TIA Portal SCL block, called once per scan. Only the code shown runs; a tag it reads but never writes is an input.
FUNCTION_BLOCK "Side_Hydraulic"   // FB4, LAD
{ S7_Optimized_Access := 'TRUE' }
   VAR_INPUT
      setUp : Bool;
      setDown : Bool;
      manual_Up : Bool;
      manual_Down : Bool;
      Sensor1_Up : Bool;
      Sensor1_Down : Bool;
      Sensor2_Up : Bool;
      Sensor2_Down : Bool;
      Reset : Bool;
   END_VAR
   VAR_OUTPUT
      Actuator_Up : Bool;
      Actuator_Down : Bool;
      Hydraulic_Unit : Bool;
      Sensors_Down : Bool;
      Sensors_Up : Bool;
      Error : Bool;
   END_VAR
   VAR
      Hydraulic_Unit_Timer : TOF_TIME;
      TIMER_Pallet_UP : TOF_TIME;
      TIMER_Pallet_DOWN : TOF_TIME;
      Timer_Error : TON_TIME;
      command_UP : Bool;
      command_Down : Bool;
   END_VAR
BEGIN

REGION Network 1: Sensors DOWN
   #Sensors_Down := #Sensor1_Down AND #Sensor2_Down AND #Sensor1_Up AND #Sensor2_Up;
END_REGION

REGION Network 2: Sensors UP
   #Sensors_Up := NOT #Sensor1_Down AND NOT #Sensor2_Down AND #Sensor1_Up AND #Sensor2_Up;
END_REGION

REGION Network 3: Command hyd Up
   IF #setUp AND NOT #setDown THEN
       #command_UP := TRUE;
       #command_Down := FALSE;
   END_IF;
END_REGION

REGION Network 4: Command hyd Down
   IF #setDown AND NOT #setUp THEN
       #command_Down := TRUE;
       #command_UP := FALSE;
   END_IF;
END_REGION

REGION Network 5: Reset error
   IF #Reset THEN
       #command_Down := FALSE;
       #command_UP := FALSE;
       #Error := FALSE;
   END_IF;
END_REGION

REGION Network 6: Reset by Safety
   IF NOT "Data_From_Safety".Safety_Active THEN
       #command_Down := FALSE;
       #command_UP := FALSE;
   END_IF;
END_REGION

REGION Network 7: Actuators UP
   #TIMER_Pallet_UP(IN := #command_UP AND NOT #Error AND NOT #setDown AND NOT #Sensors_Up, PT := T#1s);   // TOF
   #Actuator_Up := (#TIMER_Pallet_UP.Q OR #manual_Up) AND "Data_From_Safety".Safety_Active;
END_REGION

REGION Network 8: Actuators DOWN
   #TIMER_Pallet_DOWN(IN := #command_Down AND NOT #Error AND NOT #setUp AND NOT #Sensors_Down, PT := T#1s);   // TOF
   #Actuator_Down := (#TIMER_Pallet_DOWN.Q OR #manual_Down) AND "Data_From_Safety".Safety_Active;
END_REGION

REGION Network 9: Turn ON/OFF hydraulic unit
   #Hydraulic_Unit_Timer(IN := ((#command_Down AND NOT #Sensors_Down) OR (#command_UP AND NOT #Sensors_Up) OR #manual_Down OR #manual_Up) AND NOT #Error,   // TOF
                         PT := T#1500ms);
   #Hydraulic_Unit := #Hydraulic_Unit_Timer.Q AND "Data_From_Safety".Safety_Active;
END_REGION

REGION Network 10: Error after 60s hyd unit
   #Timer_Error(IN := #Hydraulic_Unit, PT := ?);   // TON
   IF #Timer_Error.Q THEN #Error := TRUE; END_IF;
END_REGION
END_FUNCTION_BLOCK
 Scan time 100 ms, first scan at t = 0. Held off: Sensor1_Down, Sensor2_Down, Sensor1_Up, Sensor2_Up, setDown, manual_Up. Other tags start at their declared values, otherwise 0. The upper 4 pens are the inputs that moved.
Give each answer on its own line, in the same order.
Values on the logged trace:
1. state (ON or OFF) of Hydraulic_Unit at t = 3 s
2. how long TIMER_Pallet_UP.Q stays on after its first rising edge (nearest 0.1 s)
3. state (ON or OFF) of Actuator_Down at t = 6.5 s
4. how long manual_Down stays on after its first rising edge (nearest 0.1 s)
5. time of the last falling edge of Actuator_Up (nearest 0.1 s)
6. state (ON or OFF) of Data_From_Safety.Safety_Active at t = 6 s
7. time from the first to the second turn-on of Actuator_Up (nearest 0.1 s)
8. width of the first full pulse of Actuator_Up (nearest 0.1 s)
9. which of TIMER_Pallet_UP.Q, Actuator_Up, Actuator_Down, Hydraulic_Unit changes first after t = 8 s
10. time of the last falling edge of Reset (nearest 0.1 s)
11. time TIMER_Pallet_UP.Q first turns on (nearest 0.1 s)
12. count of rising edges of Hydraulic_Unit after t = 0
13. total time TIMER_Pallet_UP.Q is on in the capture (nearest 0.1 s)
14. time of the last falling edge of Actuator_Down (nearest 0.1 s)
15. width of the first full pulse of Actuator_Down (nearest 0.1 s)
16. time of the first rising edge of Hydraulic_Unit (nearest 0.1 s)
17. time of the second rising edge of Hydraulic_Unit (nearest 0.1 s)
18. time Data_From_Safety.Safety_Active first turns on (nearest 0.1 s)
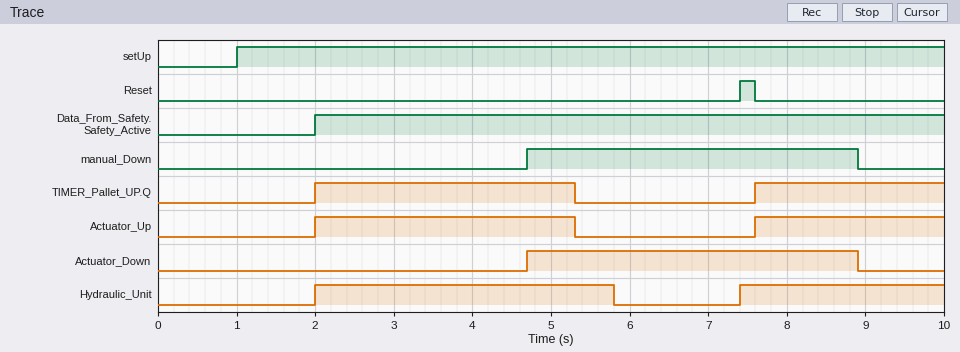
ON
3.3 s
ON
4.2 s
5.3 s
ON
5.6 s
3.3 s
Actuator_Down
7.6 s
2.0 s
2
5.7 s
8.9 s
4.2 s
2.0 s
7.4 s
2.0 s
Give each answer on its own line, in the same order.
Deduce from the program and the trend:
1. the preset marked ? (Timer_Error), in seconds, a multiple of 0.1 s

2.2 s
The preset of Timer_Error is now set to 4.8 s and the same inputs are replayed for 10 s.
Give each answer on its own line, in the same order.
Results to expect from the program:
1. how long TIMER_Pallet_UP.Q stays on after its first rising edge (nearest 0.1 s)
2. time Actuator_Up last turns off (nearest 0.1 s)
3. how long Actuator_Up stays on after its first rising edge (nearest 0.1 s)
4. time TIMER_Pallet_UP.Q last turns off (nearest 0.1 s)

5.9 s
7.9 s
5.9 s
7.9 s
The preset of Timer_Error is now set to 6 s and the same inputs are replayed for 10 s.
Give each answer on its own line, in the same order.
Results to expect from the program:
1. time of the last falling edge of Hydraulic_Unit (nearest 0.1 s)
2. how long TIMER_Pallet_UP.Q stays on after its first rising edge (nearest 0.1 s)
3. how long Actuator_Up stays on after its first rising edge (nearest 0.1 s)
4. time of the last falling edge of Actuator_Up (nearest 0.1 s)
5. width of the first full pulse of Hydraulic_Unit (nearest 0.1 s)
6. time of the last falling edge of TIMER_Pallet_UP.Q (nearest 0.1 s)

9.6 s
7.1 s
7.1 s
9.1 s
7.6 s
9.1 s
